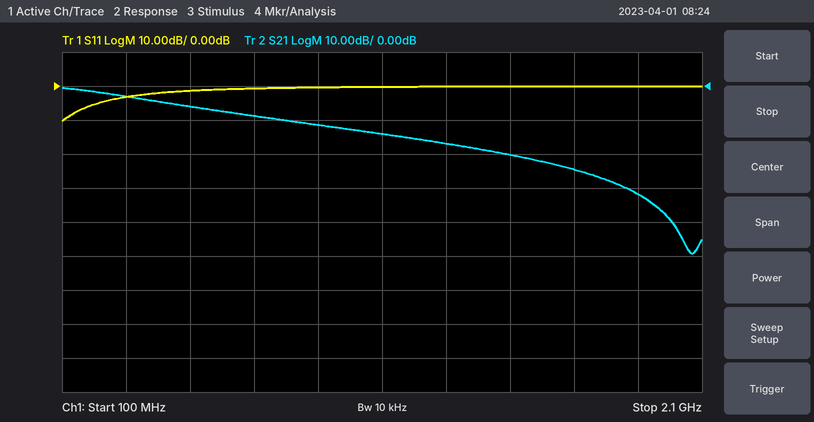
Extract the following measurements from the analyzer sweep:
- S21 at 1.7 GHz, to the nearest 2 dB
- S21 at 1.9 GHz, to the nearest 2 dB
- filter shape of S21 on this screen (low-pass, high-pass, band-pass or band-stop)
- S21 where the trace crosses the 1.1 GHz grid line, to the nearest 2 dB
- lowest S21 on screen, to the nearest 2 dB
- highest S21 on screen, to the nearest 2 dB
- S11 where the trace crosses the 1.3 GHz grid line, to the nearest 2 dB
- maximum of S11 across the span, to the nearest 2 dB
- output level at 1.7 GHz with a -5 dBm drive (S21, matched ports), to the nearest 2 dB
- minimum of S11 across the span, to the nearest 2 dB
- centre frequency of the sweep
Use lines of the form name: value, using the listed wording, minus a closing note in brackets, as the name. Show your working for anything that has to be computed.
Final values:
S21 at 1.7 GHz, to the nearest 2 dB: -24 dB
S21 at 1.9 GHz, to the nearest 2 dB: -32 dB
filter shape of S21 on this screen: low-pass
S21 where the trace crosses the 1.1 GHz grid line, to the nearest 2 dB: -14 dB
lowest S21 on screen, to the nearest 2 dB: -50 dB
highest S21 on screen, to the nearest 2 dB: 0 dB
S11 where the trace crosses the 1.3 GHz grid line, to the nearest 2 dB: 0 dB
maximum of S11 across the span, to the nearest 2 dB: 0 dB
output level at 1.7 GHz with a -5 dBm drive (S21, matched ports), to the nearest 2 dB: -5 dBm + (-24 dB) = -30 dBm
minimum of S11 across the span, to the nearest 2 dB: -10 dB
centre frequency of the sweep: 1.1 GHz
